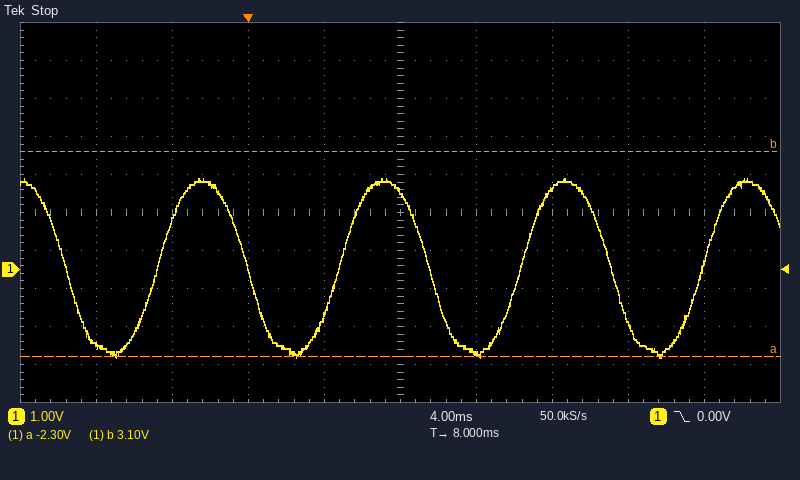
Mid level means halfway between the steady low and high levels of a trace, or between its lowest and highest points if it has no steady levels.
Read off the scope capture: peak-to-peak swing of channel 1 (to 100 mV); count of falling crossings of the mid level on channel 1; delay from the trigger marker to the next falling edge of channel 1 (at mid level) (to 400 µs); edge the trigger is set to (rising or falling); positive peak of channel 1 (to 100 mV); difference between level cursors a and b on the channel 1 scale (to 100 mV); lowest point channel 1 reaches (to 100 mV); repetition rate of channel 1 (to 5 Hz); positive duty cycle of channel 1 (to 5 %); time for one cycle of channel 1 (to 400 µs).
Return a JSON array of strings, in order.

["4.7 V", "4", "9.6 ms", "falling", "2.4 V", "5.4 V", "-2.3 V", "105 Hz", "50 %", "9.6 ms"]
